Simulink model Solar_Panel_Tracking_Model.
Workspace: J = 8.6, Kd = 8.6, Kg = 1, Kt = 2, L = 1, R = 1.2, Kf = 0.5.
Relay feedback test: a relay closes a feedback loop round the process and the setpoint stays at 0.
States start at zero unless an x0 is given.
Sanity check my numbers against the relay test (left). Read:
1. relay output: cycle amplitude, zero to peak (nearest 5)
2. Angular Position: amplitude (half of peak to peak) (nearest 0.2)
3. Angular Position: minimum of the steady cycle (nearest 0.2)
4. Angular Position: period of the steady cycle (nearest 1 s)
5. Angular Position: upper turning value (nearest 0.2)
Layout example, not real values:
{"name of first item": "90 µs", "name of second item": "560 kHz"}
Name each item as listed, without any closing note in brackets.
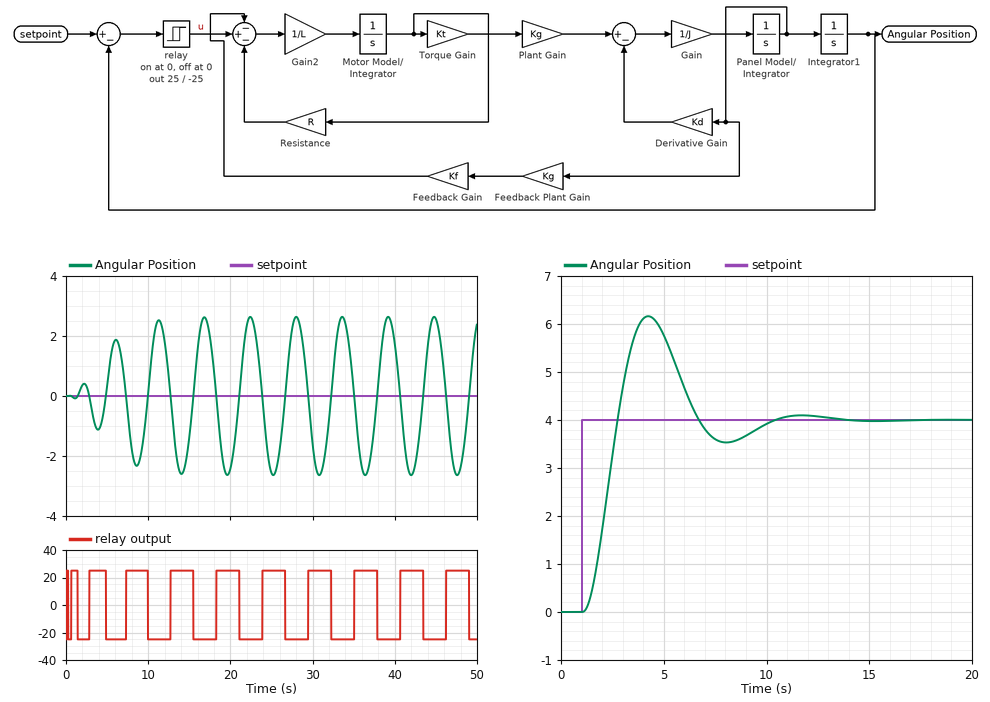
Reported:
{"relay output: cycle amplitude, zero to peak": "25", "Angular Position: amplitude (half of peak to peak)": "2.6", "Angular Position: minimum of the steady cycle": "-2.6", "Angular Position: period of the steady cycle": "6 s", "Angular Position: upper turning value": "2.6"}
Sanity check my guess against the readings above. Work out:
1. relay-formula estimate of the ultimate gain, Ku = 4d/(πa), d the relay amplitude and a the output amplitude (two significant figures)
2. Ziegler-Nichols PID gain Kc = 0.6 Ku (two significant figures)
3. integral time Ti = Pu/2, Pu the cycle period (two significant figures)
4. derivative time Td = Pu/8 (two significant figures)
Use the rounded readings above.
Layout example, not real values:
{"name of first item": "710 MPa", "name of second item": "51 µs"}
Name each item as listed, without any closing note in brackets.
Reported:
{"relay-formula estimate of the ultimate gain, Ku = 4d/(πa), d the relay amplitude and a the output amplitude": "12", "Ziegler-Nichols PID gain Kc = 0.6 Ku": "7.2", "integral time Ti = Pu/2, Pu the cycle period": "3.0 s", "derivative time Td = Pu/8": "0.75 s"}
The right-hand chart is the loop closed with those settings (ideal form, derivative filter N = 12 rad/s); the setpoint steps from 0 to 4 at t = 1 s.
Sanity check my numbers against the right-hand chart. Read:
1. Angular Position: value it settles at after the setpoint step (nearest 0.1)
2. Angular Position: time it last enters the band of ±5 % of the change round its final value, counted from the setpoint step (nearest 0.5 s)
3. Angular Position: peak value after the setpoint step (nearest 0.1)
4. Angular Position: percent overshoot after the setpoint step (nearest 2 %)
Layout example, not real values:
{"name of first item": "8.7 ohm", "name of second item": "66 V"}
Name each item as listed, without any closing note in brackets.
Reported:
{"Angular Position: value it settles at after the setpoint step": "4.0", "Angular Position: time it last enters the band of ±5 % of the change round its final value, counted from the setpoint step": "8.5 s", "Angular Position: peak value after the setpoint step": "6.2", "Angular Position: percent overshoot after the setpoint step": "54 %"}
